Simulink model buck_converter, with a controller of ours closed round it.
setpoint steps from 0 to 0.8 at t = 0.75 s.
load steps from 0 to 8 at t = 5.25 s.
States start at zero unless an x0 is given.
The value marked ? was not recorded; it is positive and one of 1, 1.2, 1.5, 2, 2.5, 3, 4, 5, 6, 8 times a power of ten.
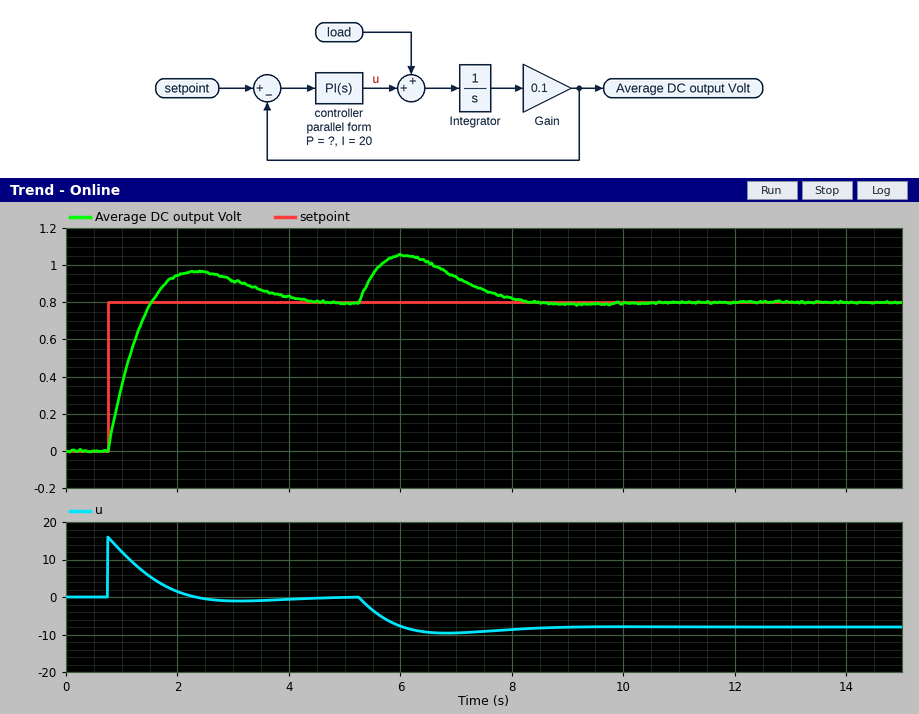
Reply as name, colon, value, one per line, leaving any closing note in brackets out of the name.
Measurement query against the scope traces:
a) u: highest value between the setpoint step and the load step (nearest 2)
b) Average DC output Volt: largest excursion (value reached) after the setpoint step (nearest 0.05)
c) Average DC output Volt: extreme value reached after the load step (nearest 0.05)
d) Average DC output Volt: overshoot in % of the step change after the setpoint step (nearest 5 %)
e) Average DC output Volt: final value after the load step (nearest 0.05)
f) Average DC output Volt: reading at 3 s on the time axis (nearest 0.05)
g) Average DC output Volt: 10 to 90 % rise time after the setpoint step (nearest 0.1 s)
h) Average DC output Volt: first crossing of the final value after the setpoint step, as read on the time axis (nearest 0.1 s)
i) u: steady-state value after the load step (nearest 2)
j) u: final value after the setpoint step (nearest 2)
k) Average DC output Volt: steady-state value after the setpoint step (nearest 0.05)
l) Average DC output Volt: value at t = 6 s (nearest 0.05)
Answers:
u: highest value between the setpoint step and the load step: 16
Average DC output Volt: largest excursion (value reached) after the setpoint step: 0.95
Average DC output Volt: extreme value reached after the load step: 1.05
Average DC output Volt: overshoot in % of the step change after the setpoint step: 20 %
Average DC output Volt: final value after the load step: 0.80
Average DC output Volt: reading at 3 s on the time axis: 0.90
Average DC output Volt: 10 to 90 % rise time after the setpoint step: 0.6 s
Average DC output Volt: first crossing of the final value after the setpoint step, as read on the time axis: 1.5 s
u: steady-state value after the load step: -8
u: final value after the setpoint step: 0
Average DC output Volt: steady-state value after the setpoint step: 0.80
Average DC output Volt: value at t = 6 s: 1.05
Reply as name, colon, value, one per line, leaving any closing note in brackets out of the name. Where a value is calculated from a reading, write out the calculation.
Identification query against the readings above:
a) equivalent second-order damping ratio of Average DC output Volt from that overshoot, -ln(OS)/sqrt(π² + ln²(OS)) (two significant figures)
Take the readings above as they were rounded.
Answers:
equivalent second-order damping ratio of Average DC output Volt from that overshoot, -ln(OS)/sqrt(π² + ln²(OS)): ln(0.2) = -1.609; 1.609 / sqrt(9.870 + 2.590) = 0.46
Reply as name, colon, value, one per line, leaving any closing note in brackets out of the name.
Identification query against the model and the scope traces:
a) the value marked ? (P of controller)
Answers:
the value marked ?: 20
